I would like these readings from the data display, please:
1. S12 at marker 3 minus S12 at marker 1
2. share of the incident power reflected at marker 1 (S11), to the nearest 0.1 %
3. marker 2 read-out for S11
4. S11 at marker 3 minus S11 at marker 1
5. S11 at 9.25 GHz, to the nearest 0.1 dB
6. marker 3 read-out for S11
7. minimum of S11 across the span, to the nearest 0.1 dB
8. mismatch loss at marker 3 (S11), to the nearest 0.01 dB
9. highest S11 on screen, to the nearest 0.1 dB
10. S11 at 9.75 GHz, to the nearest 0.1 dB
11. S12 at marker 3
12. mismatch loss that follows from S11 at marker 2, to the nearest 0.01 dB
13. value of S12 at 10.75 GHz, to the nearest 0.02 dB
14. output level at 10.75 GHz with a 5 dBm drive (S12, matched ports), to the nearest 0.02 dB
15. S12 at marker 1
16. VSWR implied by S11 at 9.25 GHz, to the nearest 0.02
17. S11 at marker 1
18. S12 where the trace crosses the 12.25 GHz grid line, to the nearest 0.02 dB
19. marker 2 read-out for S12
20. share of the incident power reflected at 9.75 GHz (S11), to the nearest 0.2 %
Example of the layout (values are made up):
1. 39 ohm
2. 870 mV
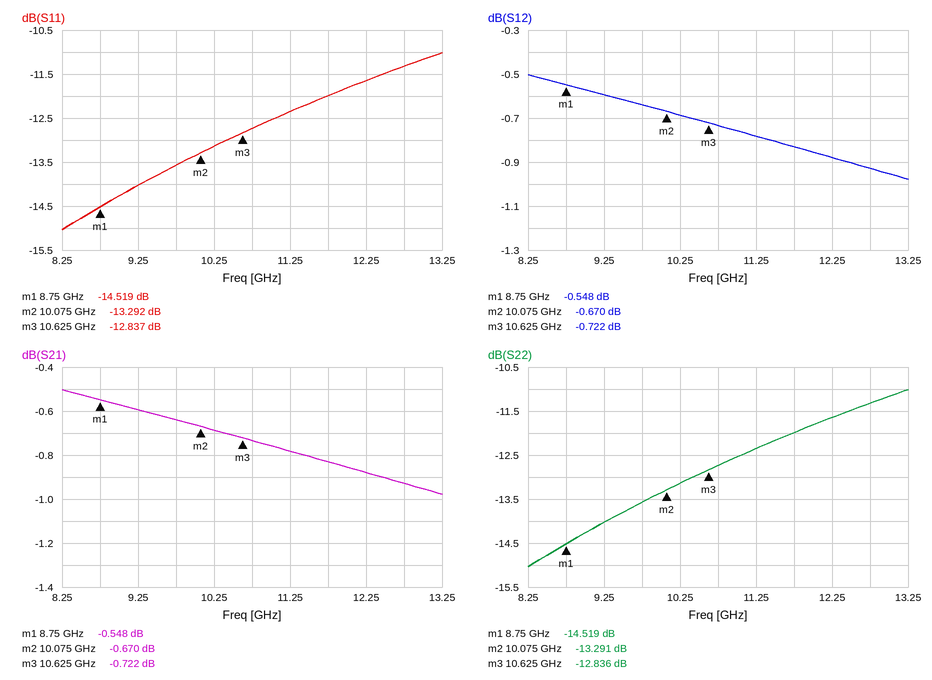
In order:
1. -0.174 dB
2. 3.5 %
3. -13.292 dB
4. 1.682 dB
5. -14.0 dB
6. -12.837 dB
7. -15.0 dB
8. 0.23 dB
9. -11.0 dB
10. -13.6 dB
11. -0.722 dB
12. 0.21 dB
13. -0.74 dB
14. 4.26 dBm
15. -0.548 dB
16. 1.50
17. -14.519 dB
18. -0.88 dB
19. -0.670 dB
20. 4.4 %
